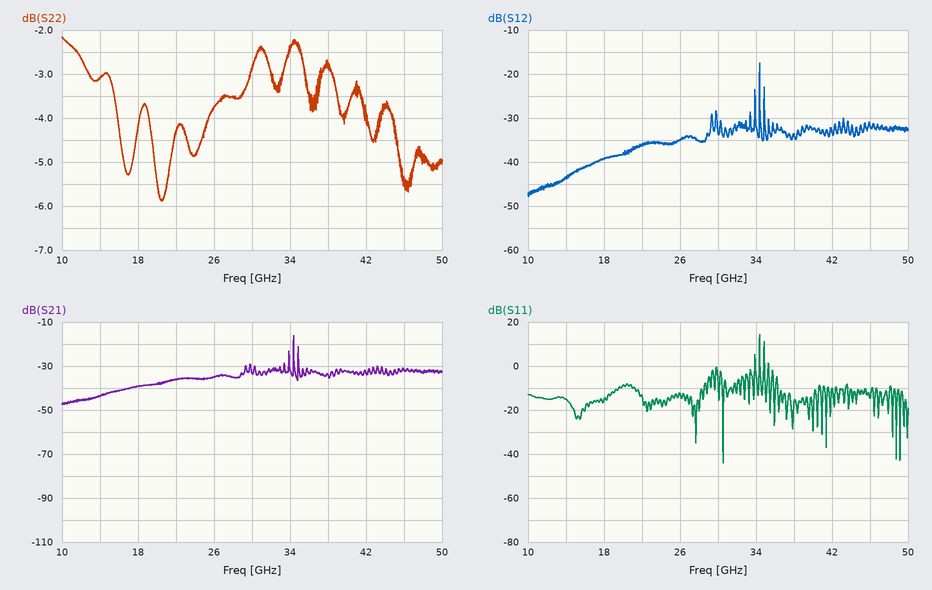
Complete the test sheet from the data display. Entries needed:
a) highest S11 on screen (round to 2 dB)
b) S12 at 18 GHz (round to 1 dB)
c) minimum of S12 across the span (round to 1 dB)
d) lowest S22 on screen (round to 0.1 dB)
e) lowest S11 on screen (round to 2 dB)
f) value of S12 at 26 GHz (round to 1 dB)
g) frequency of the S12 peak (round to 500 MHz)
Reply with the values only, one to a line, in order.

14 dB
-39 dB
-48 dB
-5.9 dB
-44 dB
-35 dB
34.5 GHz
